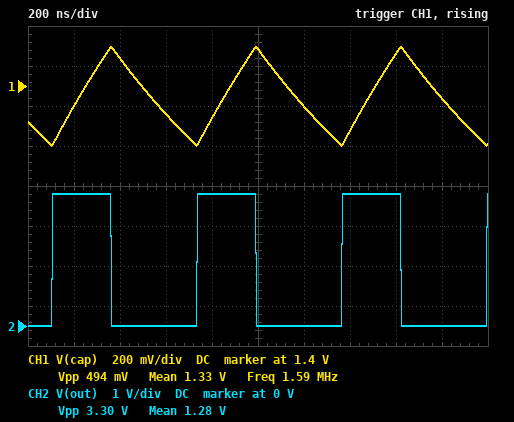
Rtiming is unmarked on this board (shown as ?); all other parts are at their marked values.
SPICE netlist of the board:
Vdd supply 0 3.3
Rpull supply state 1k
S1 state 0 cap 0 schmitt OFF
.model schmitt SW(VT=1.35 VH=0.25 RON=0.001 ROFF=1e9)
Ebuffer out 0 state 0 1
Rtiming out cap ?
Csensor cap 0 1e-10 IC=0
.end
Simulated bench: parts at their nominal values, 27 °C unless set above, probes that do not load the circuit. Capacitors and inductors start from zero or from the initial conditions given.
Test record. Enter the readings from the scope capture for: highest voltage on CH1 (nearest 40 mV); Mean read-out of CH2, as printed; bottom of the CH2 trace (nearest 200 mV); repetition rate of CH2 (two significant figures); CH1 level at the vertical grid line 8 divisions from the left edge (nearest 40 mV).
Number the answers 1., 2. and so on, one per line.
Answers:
1. 1.60 V
2. 1.28 V
3. 0 V
4. 1.6 MHz
5. 1.56 V
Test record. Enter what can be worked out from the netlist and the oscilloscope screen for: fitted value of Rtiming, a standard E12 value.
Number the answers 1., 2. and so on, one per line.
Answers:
1. 10 kΩ
